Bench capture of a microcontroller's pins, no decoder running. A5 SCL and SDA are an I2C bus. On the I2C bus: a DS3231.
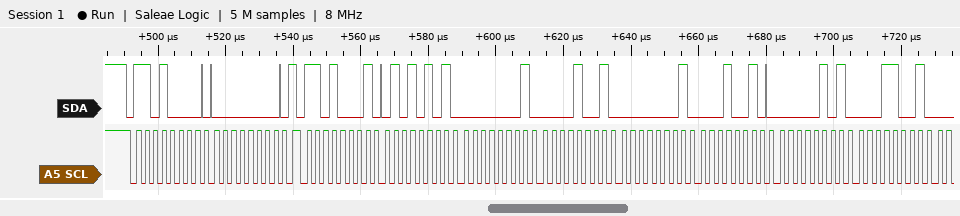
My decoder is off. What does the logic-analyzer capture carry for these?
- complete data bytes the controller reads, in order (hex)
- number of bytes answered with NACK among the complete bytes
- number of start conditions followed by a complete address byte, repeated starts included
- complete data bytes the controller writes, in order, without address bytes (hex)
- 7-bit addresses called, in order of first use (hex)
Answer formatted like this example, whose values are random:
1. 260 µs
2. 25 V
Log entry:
1. 55 01 09 01 12 05 19
2. 0
3. 2
4. 00
5. 0x68
